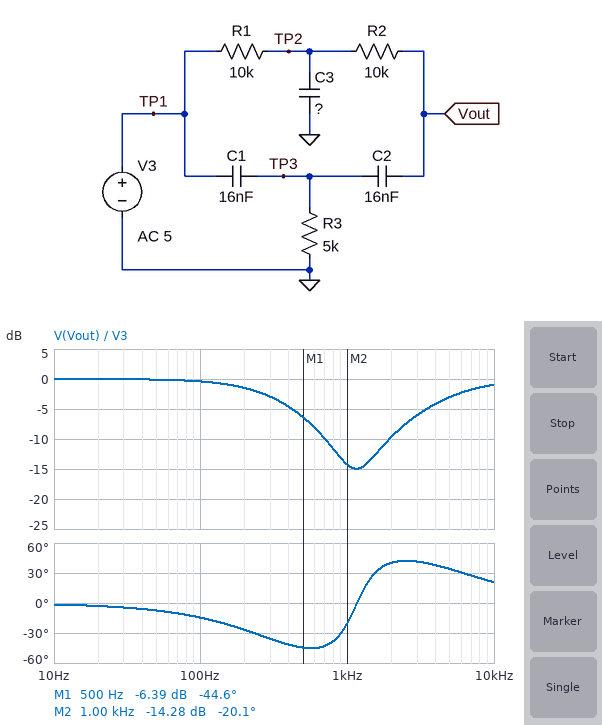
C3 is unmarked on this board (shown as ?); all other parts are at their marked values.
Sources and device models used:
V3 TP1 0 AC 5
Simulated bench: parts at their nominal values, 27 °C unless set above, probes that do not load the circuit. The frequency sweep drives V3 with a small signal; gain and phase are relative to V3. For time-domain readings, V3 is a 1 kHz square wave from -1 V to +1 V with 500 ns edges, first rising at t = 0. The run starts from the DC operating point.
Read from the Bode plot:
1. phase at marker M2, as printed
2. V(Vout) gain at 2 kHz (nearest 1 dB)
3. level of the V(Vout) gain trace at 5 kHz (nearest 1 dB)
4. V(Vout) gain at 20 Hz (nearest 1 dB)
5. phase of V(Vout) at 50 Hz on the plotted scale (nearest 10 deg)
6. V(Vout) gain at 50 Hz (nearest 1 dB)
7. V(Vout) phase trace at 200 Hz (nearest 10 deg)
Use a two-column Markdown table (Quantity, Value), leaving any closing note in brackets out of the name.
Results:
| Quantity | Value |
|---|---|
| phase at marker M2, as printed | -20.1 deg |
| V(Vout) gain at 2 kHz | -10 dB |
| level of the V(Vout) gain trace at 5 kHz | -3 dB |
| V(Vout) gain at 20 Hz | 0 dB |
| phase of V(Vout) at 50 Hz on the plotted scale | -10 deg |
| V(Vout) gain at 50 Hz | 0 dB |
| V(Vout) phase trace at 200 Hz | -30 deg |
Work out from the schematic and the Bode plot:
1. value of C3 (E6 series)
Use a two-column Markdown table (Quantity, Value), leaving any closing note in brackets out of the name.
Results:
| Quantity | Value |
|---|---|
| value of C3 | 10 nF |
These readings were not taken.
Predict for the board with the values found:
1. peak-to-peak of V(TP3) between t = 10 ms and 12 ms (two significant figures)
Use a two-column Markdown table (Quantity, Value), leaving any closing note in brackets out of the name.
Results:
| Quantity | Value |
|---|---|
| peak-to-peak of V(TP3) between t = 10 ms and 12 ms | 3.7 V |
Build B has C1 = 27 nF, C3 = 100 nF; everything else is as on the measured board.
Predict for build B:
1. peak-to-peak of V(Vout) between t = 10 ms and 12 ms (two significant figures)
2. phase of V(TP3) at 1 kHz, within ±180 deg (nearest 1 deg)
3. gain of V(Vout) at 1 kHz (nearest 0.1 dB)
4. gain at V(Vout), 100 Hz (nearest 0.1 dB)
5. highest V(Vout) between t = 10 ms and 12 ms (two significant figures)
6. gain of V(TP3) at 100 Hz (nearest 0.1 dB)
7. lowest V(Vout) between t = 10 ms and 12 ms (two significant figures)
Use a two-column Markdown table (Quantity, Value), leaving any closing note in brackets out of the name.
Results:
| Quantity | Value |
|---|---|
| peak-to-peak of V(Vout) between t = 10 ms and 12 ms | 3.9 V |
| phase of V(TP3) at 1 kHz, within ±180 deg | 45 deg |
| gain of V(Vout) at 1 kHz | -11.9 dB |
| gain at V(Vout), 100 Hz | -2.2 dB |
| highest V(Vout) between t = 10 ms and 12 ms | 1.9 V |
| gain of V(TP3) at 100 Hz | -18.7 dB |
| lowest V(Vout) between t = 10 ms and 12 ms | -1.9 V |
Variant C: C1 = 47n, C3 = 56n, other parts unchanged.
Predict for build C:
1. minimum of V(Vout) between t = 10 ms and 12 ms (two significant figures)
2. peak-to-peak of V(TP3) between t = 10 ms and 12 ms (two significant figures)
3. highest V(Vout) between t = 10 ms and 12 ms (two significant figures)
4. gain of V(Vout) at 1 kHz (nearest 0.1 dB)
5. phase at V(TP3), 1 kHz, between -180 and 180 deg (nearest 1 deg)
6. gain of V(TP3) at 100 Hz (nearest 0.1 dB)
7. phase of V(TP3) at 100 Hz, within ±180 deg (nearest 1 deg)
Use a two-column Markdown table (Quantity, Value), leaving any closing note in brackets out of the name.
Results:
| Quantity | Value |
|---|---|
| minimum of V(Vout) between t = 10 ms and 12 ms | -1.8 V |
| peak-to-peak of V(TP3) between t = 10 ms and 12 ms | 3.5 V |
| highest V(Vout) between t = 10 ms and 12 ms | 1.8 V |
| gain of V(Vout) at 1 kHz | -10.5 dB |
| phase at V(TP3), 1 kHz, between -180 and 180 deg | 32 deg |
| gain of V(TP3) at 100 Hz | -14.7 dB |
| phase of V(TP3) at 100 Hz, within ±180 deg | 72 deg |
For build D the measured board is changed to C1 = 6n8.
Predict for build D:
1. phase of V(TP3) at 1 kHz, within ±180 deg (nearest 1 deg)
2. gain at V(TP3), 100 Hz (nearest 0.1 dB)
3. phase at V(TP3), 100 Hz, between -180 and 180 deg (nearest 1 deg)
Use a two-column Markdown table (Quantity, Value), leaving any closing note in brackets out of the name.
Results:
| Quantity | Value |
|---|---|
| phase of V(TP3) at 1 kHz, within ±180 deg | 35 deg |
| gain at V(TP3), 100 Hz | -23.2 dB |
| phase at V(TP3), 100 Hz, between -180 and 180 deg | 76 deg |
